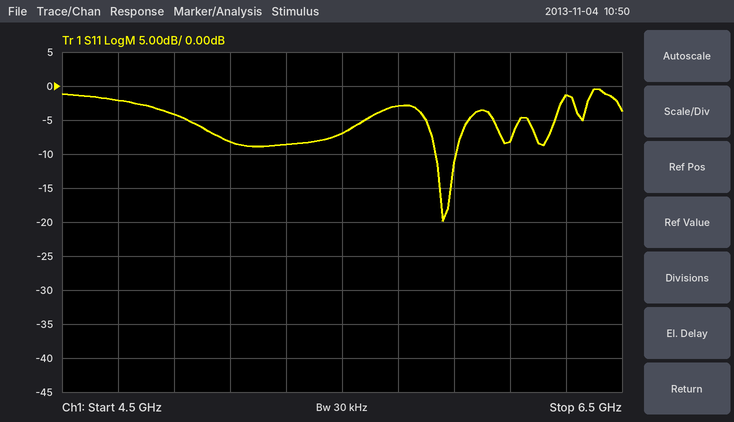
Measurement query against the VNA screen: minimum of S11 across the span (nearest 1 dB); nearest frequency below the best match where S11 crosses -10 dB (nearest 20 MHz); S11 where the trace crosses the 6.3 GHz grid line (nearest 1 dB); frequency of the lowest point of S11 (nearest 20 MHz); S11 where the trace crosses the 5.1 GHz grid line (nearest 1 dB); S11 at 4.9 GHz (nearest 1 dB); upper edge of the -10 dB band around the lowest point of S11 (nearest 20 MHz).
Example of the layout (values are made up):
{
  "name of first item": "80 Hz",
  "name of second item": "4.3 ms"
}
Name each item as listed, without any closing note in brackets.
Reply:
{
  "minimum of S11 across the span": "-20 dB",
  "nearest frequency below the best match where S11 crosses -10 dB": "5.84 GHz",
  "S11 where the trace crosses the 6.3 GHz grid line": "-1 dB",
  "frequency of the lowest point of S11": "5.86 GHz",
  "S11 where the trace crosses the 5.1 GHz grid line": "-8 dB",
  "S11 at 4.9 GHz": "-4 dB",
  "upper edge of the -10 dB band around the lowest point of S11": "5.90 GHz"
}
